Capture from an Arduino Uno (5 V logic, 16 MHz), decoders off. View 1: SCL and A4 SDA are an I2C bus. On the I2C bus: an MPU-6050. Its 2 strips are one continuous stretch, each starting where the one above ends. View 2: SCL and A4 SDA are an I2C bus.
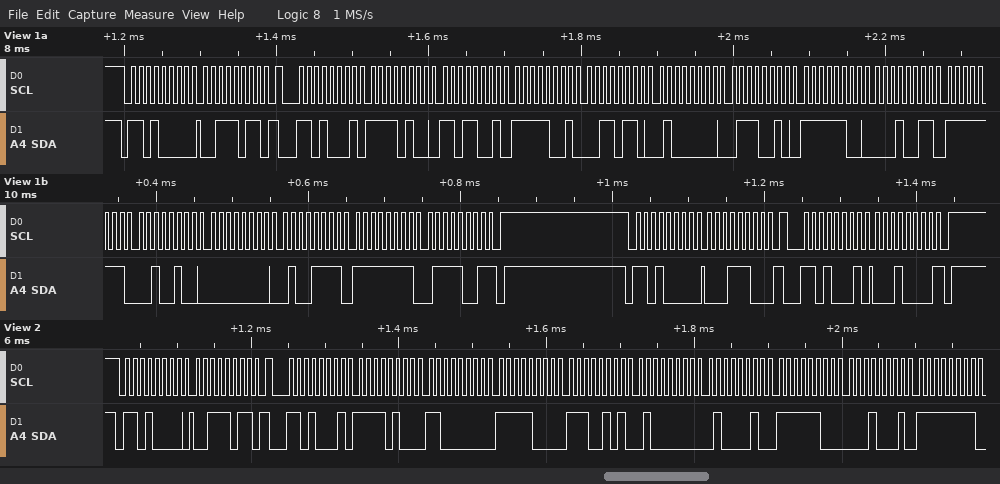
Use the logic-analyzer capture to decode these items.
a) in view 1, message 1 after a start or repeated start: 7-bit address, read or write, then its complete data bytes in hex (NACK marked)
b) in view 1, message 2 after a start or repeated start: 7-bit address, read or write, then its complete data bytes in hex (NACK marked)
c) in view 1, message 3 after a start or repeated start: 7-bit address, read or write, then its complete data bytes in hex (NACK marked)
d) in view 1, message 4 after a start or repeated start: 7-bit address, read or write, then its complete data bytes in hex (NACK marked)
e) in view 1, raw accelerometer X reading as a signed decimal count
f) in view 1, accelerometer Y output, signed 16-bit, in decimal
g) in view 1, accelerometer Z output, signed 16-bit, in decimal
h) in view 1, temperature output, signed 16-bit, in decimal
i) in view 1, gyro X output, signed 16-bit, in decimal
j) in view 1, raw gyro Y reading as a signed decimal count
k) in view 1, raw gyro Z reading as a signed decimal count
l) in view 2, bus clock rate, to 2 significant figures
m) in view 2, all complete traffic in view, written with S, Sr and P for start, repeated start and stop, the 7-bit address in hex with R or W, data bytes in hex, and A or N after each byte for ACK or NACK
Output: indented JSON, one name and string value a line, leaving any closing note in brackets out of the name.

{
  "in view 1, message 1 after a start or repeated start: 7-bit address, read or write, then its complete data bytes in hex": "0x68 write: 3B",
  "in view 1, message 2 after a start or repeated start: 7-bit address, read or write, then its complete data bytes in hex": "0x68 read: F4 D9 F9 36 40 72 FC 13 FF 24 00 4F FF 79 NACK",
  "in view 1, message 3 after a start or repeated start: 7-bit address, read or write, then its complete data bytes in hex": "0x68 write: 1C",
  "in view 1, message 4 after a start or repeated start: 7-bit address, read or write, then its complete data bytes in hex": "0x68 read: 10 NACK",
  "in view 1, raw accelerometer X reading as a signed decimal count": "-2855",
  "in view 1, accelerometer Y output, signed 16-bit, in decimal": "-1738",
  "in view 1, accelerometer Z output, signed 16-bit, in decimal": "16498",
  "in view 1, temperature output, signed 16-bit, in decimal": "-1005",
  "in view 1, gyro X output, signed 16-bit, in decimal": "-220",
  "in view 1, raw gyro Y reading as a signed decimal count": "79",
  "in view 1, raw gyro Z reading as a signed decimal count": "-135",
  "in view 2, bus clock rate, to 2 significant figures": "100 kHz",
  "in view 2, all complete traffic in view, written with S, Sr and P for start, repeated start and stop, the 7-bit address in hex with R or W, data bytes in hex, and A or N after each byte for ACK or NACK": "S 68W A 3B A Sr 68R A F4 A C0 A F8 A E5 A 40 A 42 A FC A 11 A FF A"
}
